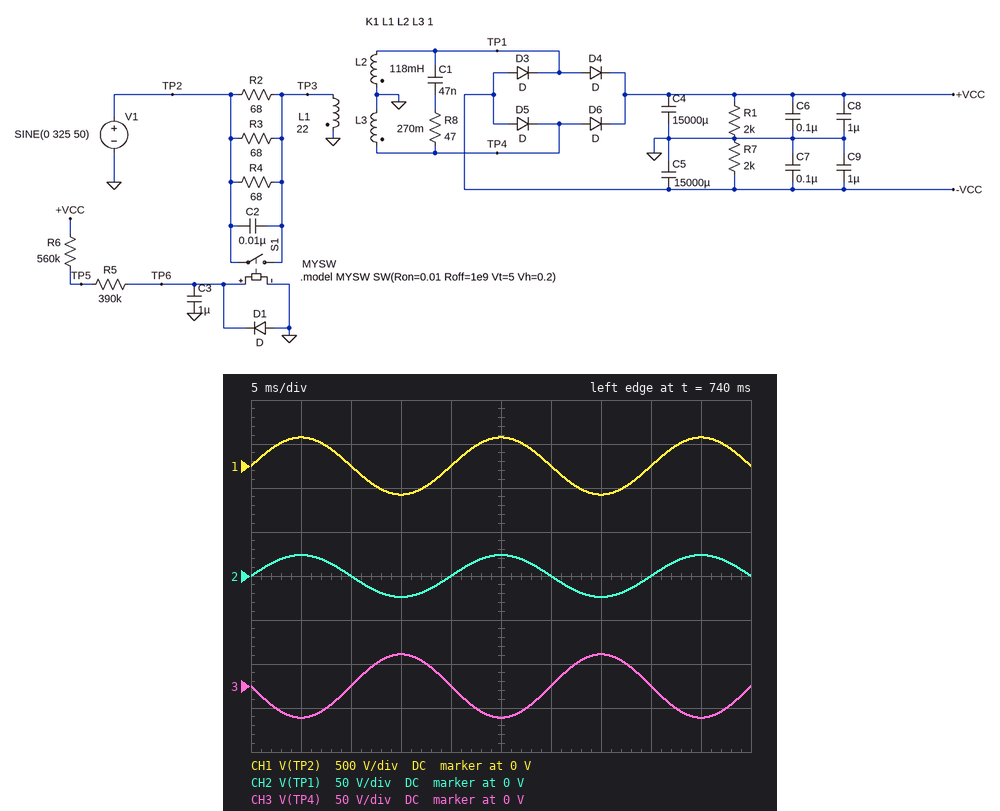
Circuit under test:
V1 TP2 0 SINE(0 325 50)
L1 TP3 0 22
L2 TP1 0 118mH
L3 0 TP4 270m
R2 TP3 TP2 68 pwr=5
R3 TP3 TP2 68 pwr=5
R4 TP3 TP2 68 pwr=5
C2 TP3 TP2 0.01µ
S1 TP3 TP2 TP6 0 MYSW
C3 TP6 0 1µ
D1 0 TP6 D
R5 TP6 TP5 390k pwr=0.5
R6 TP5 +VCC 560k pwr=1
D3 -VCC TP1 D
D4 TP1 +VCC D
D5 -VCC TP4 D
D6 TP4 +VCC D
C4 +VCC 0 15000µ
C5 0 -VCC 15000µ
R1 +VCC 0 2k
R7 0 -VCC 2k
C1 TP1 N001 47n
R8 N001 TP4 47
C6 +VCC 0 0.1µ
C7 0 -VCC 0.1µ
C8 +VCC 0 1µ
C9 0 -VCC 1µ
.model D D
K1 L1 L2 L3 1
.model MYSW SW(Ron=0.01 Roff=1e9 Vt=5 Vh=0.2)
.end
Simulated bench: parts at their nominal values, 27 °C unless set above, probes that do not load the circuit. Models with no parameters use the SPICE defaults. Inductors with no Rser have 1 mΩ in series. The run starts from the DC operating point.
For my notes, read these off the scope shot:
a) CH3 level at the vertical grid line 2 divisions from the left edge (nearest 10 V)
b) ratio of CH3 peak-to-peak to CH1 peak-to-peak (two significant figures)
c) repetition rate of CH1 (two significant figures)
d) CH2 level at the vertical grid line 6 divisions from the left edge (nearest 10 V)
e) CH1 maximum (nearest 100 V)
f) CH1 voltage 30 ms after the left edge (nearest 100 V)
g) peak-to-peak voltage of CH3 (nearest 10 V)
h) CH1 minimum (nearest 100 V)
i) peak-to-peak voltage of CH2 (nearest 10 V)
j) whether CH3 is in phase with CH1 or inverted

0 V
0.11
50 Hz
0 V
300 V
0 V
70 V
-300 V
50 V
inverted
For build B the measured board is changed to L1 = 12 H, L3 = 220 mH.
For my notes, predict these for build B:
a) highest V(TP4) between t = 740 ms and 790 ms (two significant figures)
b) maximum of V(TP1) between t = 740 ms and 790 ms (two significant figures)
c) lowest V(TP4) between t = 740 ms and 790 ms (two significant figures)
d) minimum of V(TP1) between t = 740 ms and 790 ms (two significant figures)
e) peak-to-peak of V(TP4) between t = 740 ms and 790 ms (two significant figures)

44 V
32 V
-44 V
-32 V
88 V
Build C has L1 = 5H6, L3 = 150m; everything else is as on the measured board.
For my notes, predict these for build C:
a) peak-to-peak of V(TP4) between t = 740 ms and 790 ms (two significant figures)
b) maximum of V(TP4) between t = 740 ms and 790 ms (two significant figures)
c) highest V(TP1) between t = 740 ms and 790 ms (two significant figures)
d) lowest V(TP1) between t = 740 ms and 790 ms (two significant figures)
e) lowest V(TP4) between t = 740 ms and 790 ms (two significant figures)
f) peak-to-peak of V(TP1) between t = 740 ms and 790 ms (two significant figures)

110 V
53 V
47 V
-47 V
-53 V
94 V
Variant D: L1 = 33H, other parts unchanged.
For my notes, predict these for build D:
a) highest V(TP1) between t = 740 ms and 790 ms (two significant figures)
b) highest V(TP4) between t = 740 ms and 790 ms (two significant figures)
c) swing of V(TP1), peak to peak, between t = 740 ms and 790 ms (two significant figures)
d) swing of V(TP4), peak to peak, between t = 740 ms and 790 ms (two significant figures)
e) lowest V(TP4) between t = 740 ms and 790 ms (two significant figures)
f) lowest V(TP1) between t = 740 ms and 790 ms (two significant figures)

19 V
29 V
39 V
59 V
-29 V
-19 V
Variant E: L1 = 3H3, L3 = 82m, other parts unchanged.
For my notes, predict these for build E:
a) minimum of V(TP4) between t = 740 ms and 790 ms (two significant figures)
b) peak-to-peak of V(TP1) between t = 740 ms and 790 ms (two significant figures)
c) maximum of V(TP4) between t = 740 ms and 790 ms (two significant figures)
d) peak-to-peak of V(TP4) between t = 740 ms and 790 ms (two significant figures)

-51 V
120 V
51 V
100 V
